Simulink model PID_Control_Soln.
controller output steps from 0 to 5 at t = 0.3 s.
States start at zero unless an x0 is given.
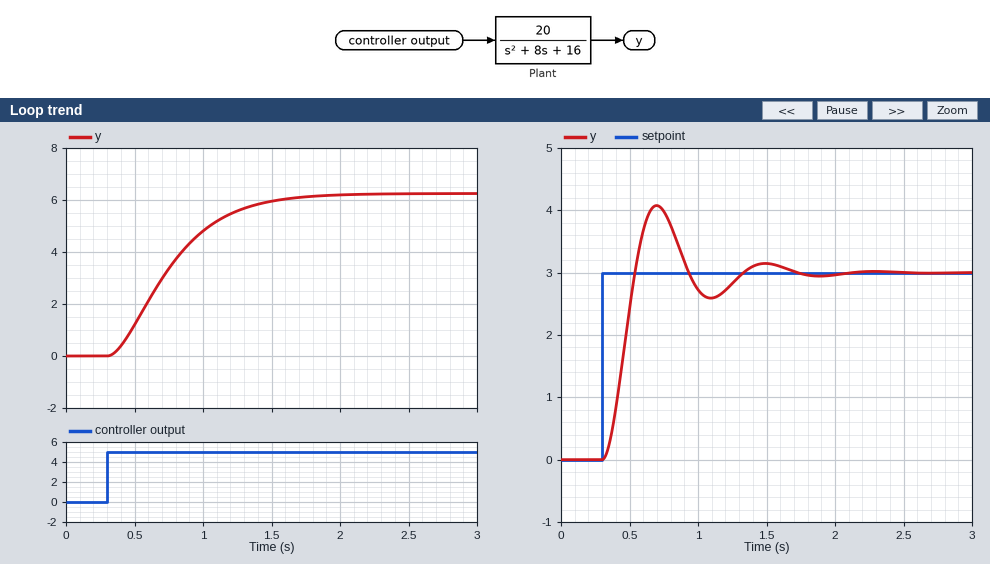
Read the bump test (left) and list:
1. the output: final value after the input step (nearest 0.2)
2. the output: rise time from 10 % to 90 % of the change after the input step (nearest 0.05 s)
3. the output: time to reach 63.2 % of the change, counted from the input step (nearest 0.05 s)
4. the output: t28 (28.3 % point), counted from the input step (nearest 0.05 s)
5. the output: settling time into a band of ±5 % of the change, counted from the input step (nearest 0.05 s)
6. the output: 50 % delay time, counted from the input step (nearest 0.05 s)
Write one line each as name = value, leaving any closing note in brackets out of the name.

the output: final value after the input step = 6.2
the output: rise time from 10 % to 90 % of the change after the input step = 0.85 s
the output: time to reach 63.2 % of the change, counted from the input step = 0.55 s
the output: t28 (28.3 % point), counted from the input step = 0.25 s
the output: settling time into a band of ±5 % of the change, counted from the input step = 1.20 s
the output: 50 % delay time, counted from the input step = 0.40 s
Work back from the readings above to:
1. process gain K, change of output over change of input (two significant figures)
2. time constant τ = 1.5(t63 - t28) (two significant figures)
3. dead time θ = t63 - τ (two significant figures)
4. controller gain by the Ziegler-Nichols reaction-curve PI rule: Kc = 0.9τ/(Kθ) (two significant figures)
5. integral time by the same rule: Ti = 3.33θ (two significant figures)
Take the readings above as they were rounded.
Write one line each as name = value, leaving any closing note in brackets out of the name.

process gain K, change of output over change of input = 1.2
time constant τ = 1.5(t63 - t28) = 0.45 s
dead time θ = t63 - τ = 0.10 s
controller gain by the Ziegler-Nichols reaction-curve PI rule: Kc = 0.9τ/(Kθ) = 3.4
integral time by the same rule: Ti = 3.33θ = 0.33 s
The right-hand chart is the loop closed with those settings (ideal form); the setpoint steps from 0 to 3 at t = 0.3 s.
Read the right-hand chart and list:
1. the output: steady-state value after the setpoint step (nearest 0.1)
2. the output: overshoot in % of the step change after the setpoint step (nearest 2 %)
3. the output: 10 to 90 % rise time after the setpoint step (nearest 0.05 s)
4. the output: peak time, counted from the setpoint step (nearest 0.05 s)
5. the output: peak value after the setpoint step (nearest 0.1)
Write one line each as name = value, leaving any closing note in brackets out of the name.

the output: steady-state value after the setpoint step = 3.0
the output: overshoot in % of the step change after the setpoint step = 36 %
the output: 10 to 90 % rise time after the setpoint step = 0.15 s
the output: peak time, counted from the setpoint step = 0.40 s
the output: peak value after the setpoint step = 4.1
